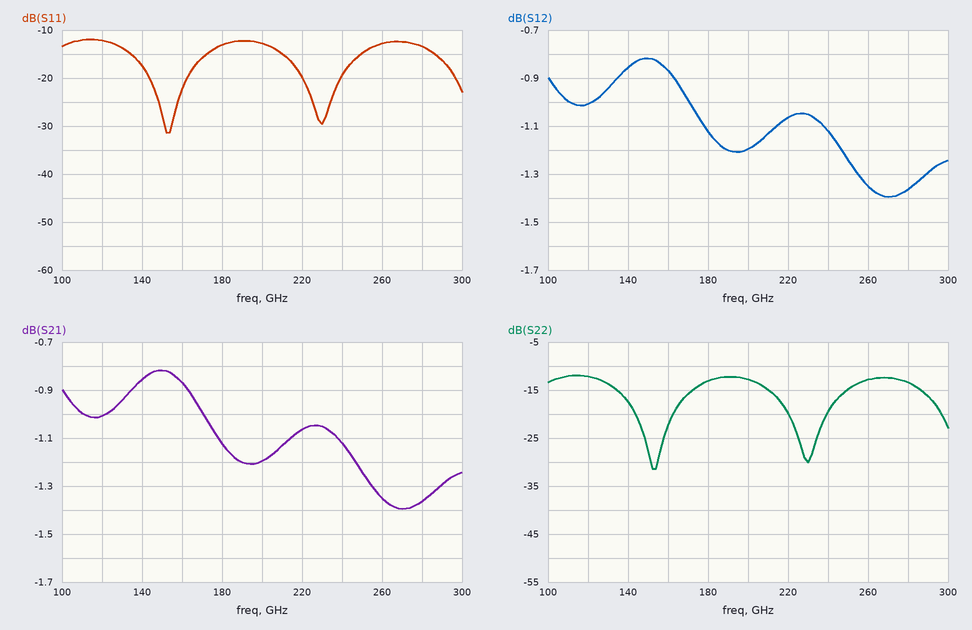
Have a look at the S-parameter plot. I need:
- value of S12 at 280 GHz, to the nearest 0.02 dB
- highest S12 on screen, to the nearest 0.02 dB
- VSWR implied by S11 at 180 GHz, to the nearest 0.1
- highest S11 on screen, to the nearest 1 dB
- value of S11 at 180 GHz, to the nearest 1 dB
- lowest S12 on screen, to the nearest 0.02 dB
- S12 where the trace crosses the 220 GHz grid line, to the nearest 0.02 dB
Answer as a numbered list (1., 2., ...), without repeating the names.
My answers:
1. -1.36 dB
2. -0.82 dB
3. 1.6
4. -12 dB
5. -13 dB
6. -1.40 dB
7. -1.06 dB
